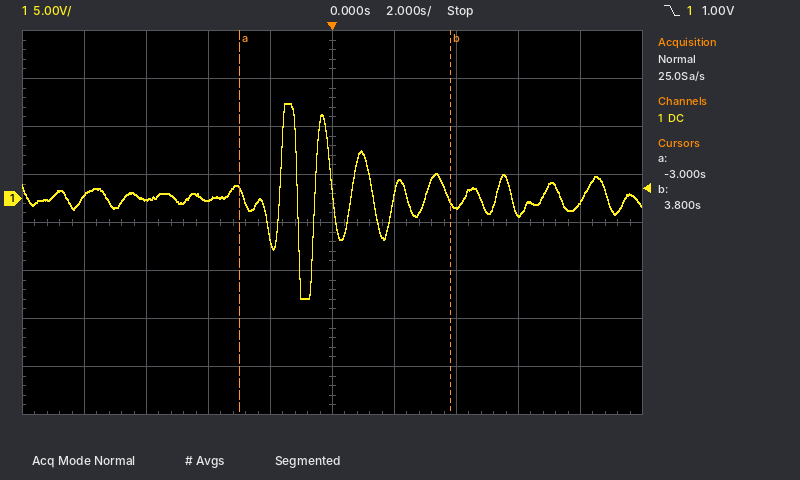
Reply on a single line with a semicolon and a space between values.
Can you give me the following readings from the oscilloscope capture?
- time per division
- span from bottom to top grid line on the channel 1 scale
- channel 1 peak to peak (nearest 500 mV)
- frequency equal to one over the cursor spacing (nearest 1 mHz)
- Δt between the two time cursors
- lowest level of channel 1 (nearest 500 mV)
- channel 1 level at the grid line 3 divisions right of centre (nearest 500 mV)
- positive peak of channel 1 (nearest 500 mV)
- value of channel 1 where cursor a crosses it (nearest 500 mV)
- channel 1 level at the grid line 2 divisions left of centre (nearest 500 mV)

2 s; 40 V; 20.5 V; 147 mHz; 6.8 s; -10.5 V; -1.5 V; 10.0 V; 1.0 V; 0.0 V
